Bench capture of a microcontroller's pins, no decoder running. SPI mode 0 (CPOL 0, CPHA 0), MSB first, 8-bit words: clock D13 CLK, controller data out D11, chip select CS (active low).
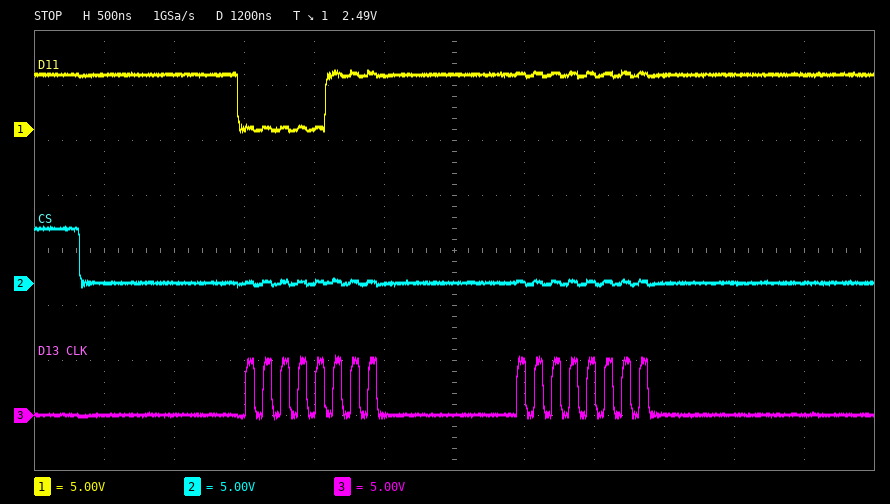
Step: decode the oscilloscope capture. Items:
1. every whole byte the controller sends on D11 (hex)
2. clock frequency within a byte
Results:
0x07 0xFF
8 MHz
